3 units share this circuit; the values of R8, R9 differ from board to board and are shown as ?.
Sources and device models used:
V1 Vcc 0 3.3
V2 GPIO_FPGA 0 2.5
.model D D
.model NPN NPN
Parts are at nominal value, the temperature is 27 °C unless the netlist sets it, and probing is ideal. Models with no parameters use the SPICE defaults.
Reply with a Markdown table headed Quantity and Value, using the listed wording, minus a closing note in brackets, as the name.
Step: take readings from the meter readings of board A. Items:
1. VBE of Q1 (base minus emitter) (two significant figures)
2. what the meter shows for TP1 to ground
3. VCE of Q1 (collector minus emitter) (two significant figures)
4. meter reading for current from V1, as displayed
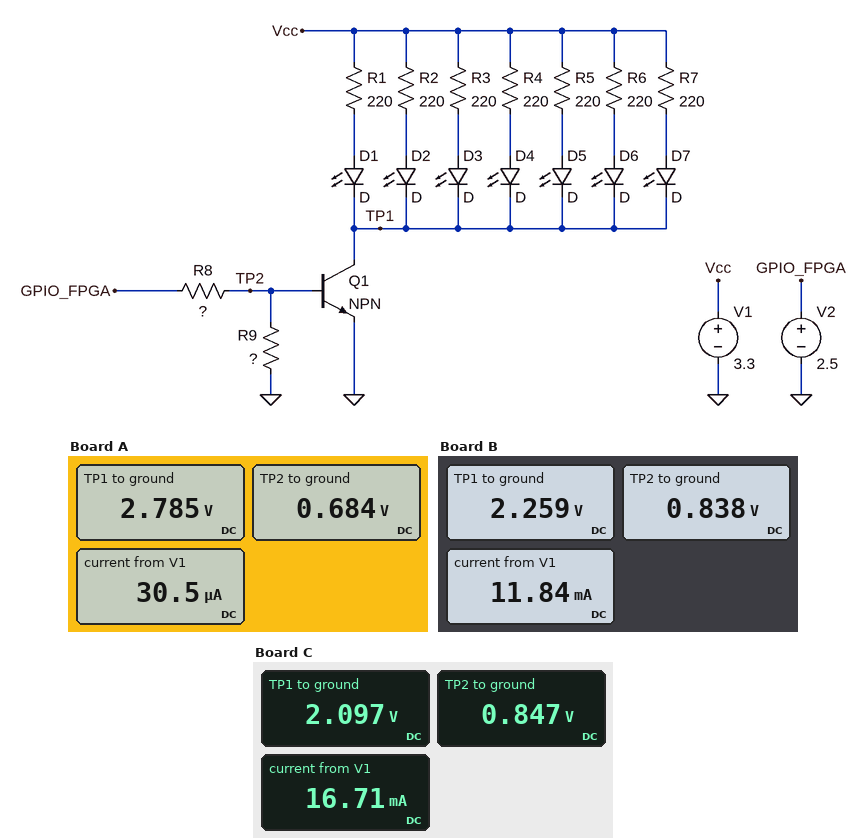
| Quantity | Value |
|---|---|
| VBE of Q1 (base minus emitter) | 680 mV |
| what the meter shows for TP1 to ground | 2.785 V |
| VCE of Q1 (collector minus emitter) | 2.8 V |
| meter reading for current from V1, as displayed | 30.5 µA |
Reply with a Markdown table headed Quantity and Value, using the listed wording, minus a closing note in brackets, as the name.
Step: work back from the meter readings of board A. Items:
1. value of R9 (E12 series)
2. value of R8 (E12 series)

| Quantity | Value |
|---|---|
| value of R9 | 6.8 kΩ |
| value of R8 | 18 kΩ |
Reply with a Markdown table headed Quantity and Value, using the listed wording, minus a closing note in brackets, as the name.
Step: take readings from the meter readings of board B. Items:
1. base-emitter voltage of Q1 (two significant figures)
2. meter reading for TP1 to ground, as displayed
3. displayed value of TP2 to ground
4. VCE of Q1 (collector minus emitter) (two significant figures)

| Quantity | Value |
|---|---|
| base-emitter voltage of Q1 | 840 mV |
| meter reading for TP1 to ground, as displayed | 2.259 V |
| displayed value of TP2 to ground | 0.838 V |
| VCE of Q1 (collector minus emitter) | 2.3 V |
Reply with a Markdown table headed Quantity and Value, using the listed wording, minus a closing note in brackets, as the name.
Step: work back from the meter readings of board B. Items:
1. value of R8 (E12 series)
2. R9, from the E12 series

| Quantity | Value |
|---|---|
| value of R8 | 5.6 kΩ |
| R9, from the E12 series | 4.7 kΩ |
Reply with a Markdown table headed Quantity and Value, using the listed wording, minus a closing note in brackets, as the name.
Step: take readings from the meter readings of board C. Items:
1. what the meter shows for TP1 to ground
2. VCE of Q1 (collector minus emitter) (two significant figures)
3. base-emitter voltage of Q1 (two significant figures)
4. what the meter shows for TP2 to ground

| Quantity | Value |
|---|---|
| what the meter shows for TP1 to ground | 2.097 V |
| VCE of Q1 (collector minus emitter) | 2.1 V |
| base-emitter voltage of Q1 | 850 mV |
| what the meter shows for TP2 to ground | 0.847 V |
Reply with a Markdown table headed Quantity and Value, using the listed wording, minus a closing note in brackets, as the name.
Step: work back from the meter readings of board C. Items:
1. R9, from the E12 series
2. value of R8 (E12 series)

| Quantity | Value |
|---|---|
| R9, from the E12 series | 3.3 kΩ |
| value of R8 | 3.9 kΩ |
